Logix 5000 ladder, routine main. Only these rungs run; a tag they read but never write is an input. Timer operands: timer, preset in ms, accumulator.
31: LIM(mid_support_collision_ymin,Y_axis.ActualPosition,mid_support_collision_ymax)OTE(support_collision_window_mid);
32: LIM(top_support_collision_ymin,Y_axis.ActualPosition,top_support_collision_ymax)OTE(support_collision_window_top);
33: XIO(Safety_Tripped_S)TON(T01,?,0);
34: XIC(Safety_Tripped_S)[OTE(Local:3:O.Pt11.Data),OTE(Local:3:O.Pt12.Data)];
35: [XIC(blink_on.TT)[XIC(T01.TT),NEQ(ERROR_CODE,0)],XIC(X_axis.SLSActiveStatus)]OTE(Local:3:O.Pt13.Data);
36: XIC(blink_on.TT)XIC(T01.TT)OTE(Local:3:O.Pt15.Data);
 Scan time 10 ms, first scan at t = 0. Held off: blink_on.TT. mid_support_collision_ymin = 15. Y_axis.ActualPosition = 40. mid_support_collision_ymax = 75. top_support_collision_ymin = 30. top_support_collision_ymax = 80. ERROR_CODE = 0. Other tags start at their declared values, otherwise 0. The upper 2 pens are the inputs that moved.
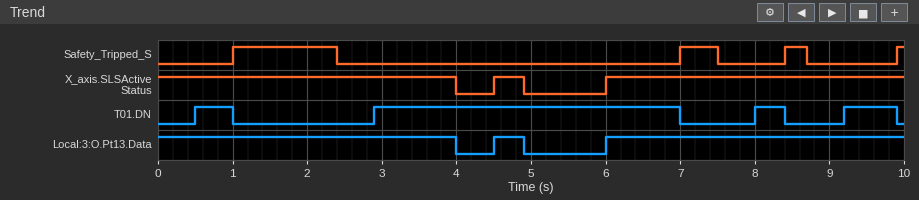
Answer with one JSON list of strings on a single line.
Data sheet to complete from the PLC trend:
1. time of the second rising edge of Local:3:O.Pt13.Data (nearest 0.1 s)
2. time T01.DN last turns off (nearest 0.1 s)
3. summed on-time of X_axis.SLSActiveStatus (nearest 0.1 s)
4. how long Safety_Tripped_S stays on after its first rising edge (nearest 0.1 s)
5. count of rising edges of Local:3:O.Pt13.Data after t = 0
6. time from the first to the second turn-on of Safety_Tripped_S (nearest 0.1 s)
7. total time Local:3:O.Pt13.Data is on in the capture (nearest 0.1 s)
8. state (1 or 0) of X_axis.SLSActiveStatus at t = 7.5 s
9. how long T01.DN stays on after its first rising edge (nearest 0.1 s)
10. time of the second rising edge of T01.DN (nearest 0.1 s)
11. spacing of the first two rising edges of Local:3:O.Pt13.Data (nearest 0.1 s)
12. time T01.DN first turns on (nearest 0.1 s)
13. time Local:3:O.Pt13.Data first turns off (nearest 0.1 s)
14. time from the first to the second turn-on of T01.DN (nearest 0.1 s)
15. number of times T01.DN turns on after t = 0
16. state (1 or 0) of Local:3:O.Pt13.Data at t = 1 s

["6.0 s", "9.9 s", "8.4 s", "1.4 s", "2", "6.0 s", "8.4 s", "1", "0.5 s", "2.9 s", "1.5 s", "0.5 s", "4.0 s", "2.4 s", "4", "1"]
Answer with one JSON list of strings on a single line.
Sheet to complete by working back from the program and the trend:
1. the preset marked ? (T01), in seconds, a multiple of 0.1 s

["0.5 s"]
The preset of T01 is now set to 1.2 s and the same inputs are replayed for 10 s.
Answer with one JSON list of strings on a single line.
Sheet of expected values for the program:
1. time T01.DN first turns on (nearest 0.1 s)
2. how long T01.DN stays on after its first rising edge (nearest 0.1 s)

["3.6 s", "3.4 s"]
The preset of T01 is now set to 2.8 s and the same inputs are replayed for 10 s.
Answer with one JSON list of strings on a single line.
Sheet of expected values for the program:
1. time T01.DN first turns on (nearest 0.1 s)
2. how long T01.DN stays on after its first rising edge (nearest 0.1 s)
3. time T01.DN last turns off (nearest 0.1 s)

["5.2 s", "1.8 s", "7.0 s"]
